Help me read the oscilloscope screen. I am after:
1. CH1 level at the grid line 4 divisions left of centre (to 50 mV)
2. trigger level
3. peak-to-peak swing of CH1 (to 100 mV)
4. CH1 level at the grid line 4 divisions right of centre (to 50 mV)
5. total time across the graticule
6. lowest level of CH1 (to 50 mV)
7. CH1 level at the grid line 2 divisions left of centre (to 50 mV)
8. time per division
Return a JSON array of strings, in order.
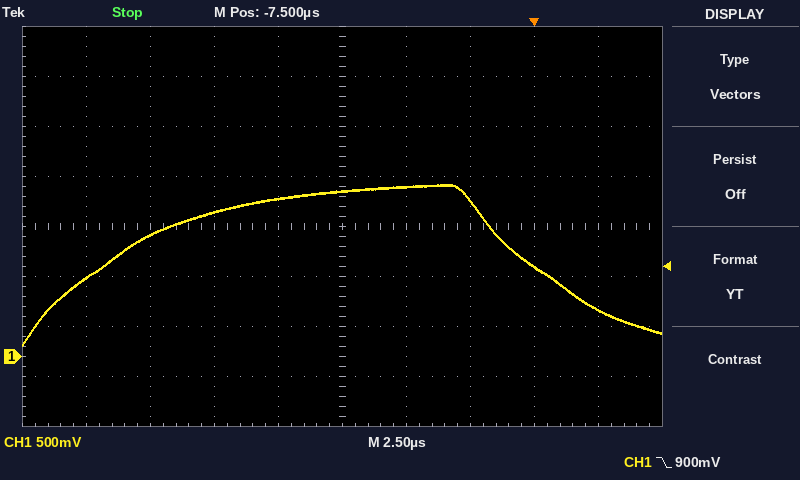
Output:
["800 mV", "900 mV", "1.60 V", "450 mV", "25 µs", "100 mV", "1.45 V", "2.5 µs"]
